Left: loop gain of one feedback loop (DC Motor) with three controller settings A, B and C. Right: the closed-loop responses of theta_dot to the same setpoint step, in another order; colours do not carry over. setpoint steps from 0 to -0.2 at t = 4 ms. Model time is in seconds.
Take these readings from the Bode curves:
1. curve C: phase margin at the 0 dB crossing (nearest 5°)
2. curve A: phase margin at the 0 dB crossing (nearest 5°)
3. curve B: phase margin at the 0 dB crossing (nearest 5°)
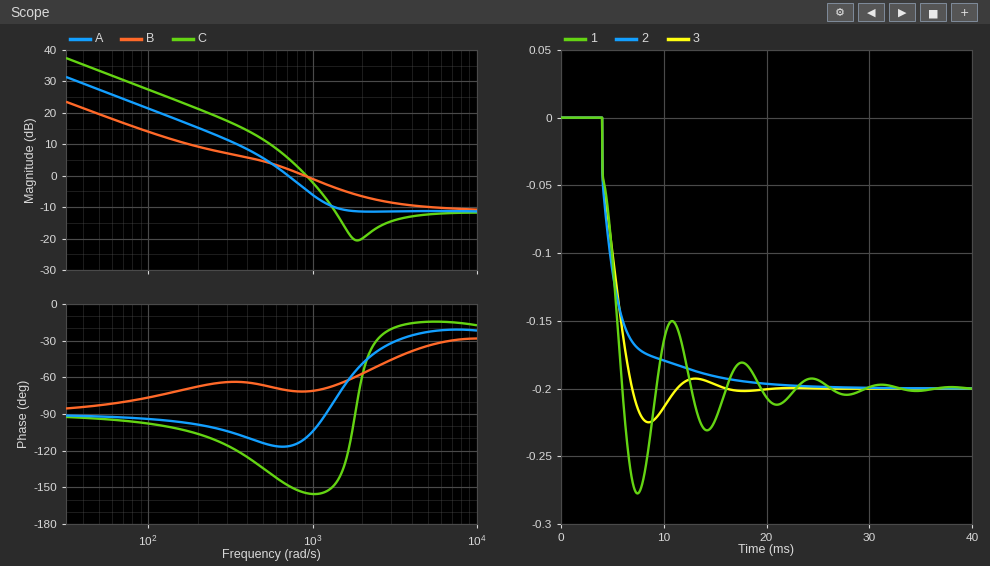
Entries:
25°
65°
110°
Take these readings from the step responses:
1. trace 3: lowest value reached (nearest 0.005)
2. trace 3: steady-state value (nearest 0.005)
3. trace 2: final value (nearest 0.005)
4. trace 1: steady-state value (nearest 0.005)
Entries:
-0.225
-0.200
-0.200
-0.200
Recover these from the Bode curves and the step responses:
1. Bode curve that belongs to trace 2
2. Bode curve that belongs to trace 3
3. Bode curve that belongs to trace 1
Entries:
B
A
C
